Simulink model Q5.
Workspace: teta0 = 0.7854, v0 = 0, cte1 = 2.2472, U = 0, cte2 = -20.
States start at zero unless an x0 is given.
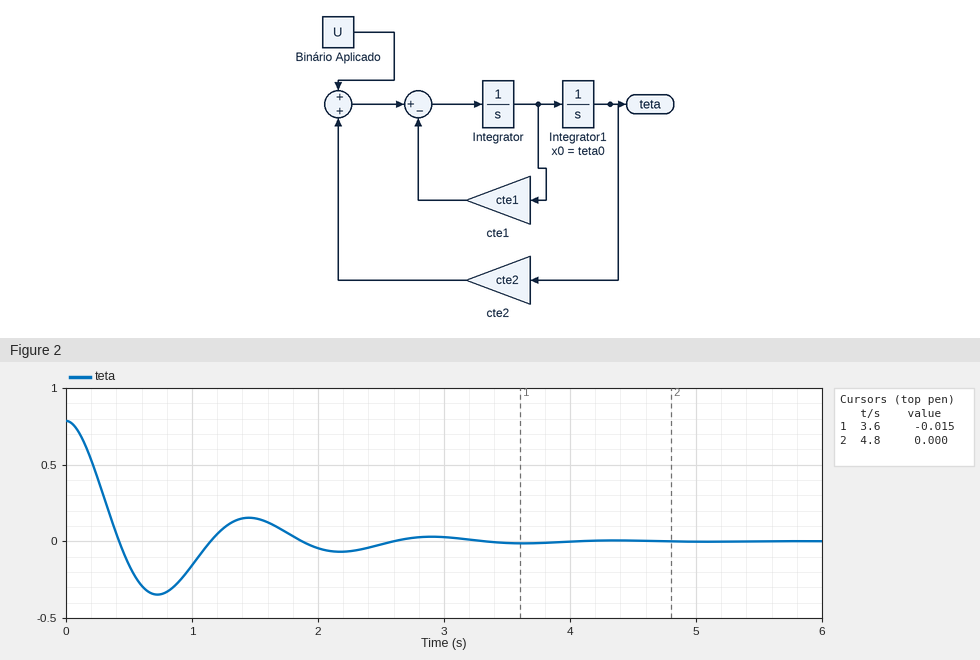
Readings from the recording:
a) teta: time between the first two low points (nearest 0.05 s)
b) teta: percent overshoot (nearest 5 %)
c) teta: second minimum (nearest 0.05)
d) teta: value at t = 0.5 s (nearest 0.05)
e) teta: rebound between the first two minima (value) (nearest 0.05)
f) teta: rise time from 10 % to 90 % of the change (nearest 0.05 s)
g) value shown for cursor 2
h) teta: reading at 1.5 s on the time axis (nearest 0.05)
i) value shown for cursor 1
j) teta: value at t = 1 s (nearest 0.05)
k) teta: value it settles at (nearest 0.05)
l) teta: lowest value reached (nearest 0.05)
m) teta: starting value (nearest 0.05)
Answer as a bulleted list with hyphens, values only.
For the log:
- 1.45 s
- 45 %
- -0.05
- -0.15
- 0.15
- 0.30 s
- 0.000
- 0.15
- -0.015
- -0.15
- 0.00
- -0.35
- 0.80
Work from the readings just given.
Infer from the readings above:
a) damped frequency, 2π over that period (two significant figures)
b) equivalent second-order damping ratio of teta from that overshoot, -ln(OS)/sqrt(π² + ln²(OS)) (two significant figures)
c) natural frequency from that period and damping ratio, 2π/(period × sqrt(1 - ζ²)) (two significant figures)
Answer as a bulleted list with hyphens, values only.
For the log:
- 4.3 rad/s
- 0.25
- 4.5 rad/s
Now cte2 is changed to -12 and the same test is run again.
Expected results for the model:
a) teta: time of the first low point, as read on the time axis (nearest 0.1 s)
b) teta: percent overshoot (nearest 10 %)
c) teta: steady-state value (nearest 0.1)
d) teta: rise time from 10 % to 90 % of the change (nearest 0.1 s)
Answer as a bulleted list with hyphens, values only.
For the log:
- 1.0 s
- 30 %
- 0.0
- 0.4 s
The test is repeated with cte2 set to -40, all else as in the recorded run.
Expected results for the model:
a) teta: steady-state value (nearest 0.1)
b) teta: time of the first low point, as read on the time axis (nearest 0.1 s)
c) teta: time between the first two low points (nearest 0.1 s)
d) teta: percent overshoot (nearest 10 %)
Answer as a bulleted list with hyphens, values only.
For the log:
- 0.0
- 0.5 s
- 1.0 s
- 60 %
